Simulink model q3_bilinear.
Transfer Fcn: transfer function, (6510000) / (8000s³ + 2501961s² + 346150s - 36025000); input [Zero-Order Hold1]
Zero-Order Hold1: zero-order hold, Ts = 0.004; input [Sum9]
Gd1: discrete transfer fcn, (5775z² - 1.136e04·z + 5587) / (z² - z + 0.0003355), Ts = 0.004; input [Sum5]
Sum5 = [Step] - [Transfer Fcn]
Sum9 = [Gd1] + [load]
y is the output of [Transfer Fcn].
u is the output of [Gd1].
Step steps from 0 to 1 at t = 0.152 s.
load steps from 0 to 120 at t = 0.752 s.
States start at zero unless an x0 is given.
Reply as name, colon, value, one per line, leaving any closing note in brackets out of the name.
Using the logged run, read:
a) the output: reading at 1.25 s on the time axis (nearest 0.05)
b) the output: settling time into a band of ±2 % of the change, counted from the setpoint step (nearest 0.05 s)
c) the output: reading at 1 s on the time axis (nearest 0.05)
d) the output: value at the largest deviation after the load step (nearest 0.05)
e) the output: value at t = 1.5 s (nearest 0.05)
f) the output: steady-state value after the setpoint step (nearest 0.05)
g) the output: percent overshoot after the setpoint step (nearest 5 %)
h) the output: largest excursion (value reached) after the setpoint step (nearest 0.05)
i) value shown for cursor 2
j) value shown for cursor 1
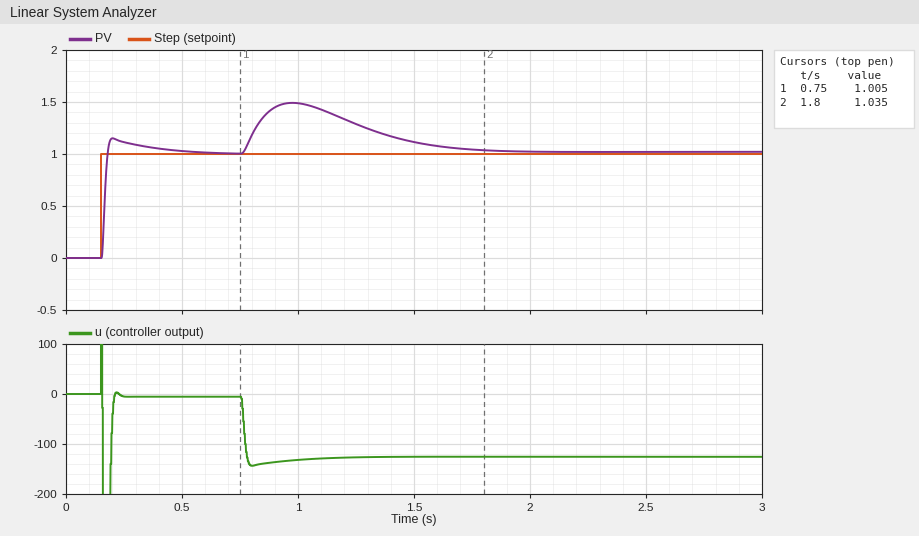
the output: reading at 1.25 s on the time axis: 1.30
the output: settling time into a band of ±2 % of the change, counted from the setpoint step: 0.40 s
the output: reading at 1 s on the time axis: 1.50
the output: value at the largest deviation after the load step: 1.50
the output: value at t = 1.5 s: 1.10
the output: steady-state value after the setpoint step: 1.00
the output: percent overshoot after the setpoint step: 15 %
the output: largest excursion (value reached) after the setpoint step: 1.15
value shown for cursor 2: 1.035
value shown for cursor 1: 1.005
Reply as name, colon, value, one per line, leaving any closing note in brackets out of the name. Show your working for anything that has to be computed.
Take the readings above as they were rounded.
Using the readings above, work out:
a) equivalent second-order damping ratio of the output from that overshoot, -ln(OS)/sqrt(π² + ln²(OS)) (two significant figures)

equivalent second-order damping ratio of the output from that overshoot, -ln(OS)/sqrt(π² + ln²(OS)): ln(0.15) = -1.897; 1.897 / sqrt(9.870 + 3.599) = 0.52
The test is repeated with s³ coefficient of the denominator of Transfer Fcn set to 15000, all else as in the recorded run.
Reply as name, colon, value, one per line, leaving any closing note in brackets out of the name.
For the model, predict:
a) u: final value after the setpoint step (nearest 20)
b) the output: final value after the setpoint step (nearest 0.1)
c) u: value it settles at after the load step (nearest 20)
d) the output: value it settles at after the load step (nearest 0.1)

u: final value after the setpoint step: 0
the output: final value after the setpoint step: 1.0
u: value it settles at after the load step: -120
the output: value it settles at after the load step: 1.0
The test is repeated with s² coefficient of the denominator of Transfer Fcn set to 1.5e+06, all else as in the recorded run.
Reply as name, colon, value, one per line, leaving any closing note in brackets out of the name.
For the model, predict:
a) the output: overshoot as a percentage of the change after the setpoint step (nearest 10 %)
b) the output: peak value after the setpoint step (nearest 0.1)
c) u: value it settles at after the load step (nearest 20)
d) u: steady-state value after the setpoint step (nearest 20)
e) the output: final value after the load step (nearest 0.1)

the output: overshoot as a percentage of the change after the setpoint step: 40 %
the output: peak value after the setpoint step: 1.4
u: value it settles at after the load step: -120
u: steady-state value after the setpoint step: 0
the output: final value after the load step: 1.0
